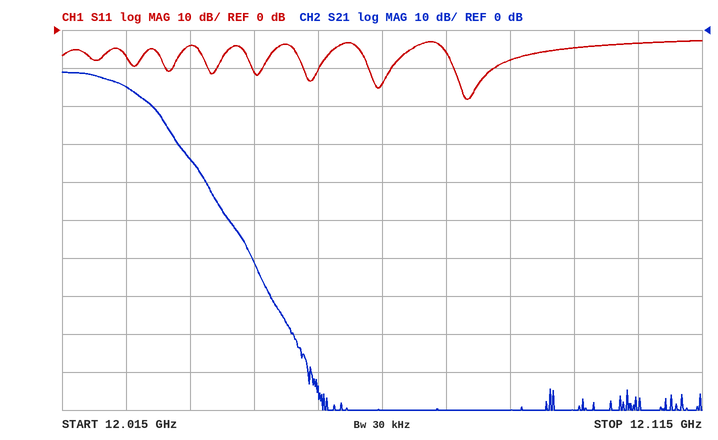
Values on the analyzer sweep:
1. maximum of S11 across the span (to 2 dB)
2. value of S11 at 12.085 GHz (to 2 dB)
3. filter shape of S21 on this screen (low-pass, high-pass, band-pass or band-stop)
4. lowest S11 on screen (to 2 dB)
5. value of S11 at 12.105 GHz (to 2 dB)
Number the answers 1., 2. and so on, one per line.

1. -2 dB
2. -8 dB
3. low-pass
4. -18 dB
5. -4 dB
